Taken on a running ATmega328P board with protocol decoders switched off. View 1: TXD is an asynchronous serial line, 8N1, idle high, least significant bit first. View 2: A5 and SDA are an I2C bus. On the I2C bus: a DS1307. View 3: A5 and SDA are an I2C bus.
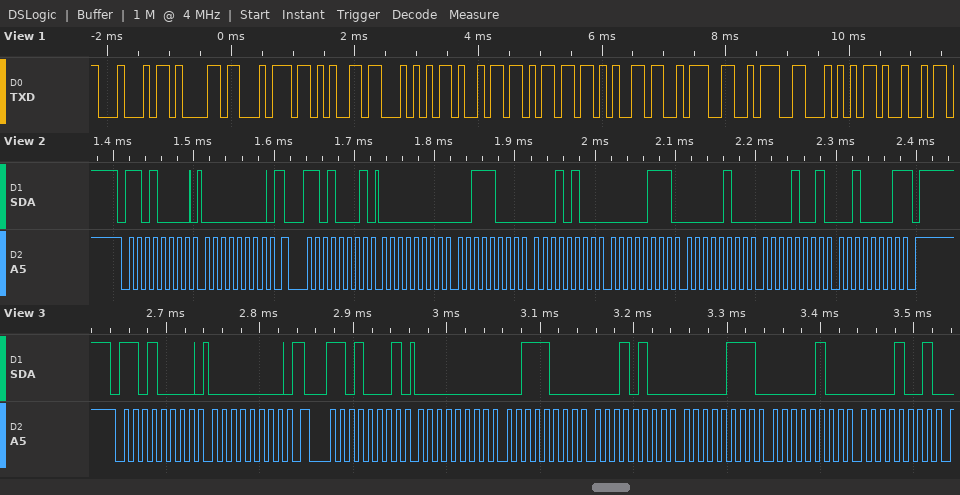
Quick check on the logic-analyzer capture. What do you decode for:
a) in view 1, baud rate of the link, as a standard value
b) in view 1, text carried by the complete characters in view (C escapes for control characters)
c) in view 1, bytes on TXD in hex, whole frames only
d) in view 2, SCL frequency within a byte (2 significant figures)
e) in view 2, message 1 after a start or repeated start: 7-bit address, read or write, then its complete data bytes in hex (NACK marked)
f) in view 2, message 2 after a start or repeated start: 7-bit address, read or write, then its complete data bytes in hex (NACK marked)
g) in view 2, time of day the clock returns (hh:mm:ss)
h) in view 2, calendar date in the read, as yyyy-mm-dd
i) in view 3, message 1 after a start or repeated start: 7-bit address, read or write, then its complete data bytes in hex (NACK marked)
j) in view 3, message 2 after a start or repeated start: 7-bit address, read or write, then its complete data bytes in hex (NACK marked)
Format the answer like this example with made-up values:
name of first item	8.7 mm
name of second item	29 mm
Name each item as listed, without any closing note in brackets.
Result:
in view 1, baud rate of the link, as a standard value	9600 baud
in view 1, text carried by the complete characters in view	"DateTime::TI"
in view 1, bytes on TXD in hex, whole frames only	0x44 0x61 0x74 0x65 0x54 0x69 0x6D 0x65 0x3A 0x3A 0x54 0x49
in view 2, SCL frequency within a byte	100 kHz
in view 2, message 1 after a start or repeated start: 7-bit address, read or write, then its complete data bytes in hex	0x68 write: 00
in view 2, message 2 after a start or repeated start: 7-bit address, read or write, then its complete data bytes in hex	0x68 read: 00 38 14 07 04 09 21 NACK
in view 2, time of day the clock returns	14:38:00
in view 2, calendar date in the read, as yyyy-mm-dd	2021-09-04
in view 3, message 1 after a start or repeated start: 7-bit address, read or write, then its complete data bytes in hex	0x68 write: 00
in view 3, message 2 after a start or repeated start: 7-bit address, read or write, then its complete data bytes in hex	0x68 read: 00 38 14 07 04 09
